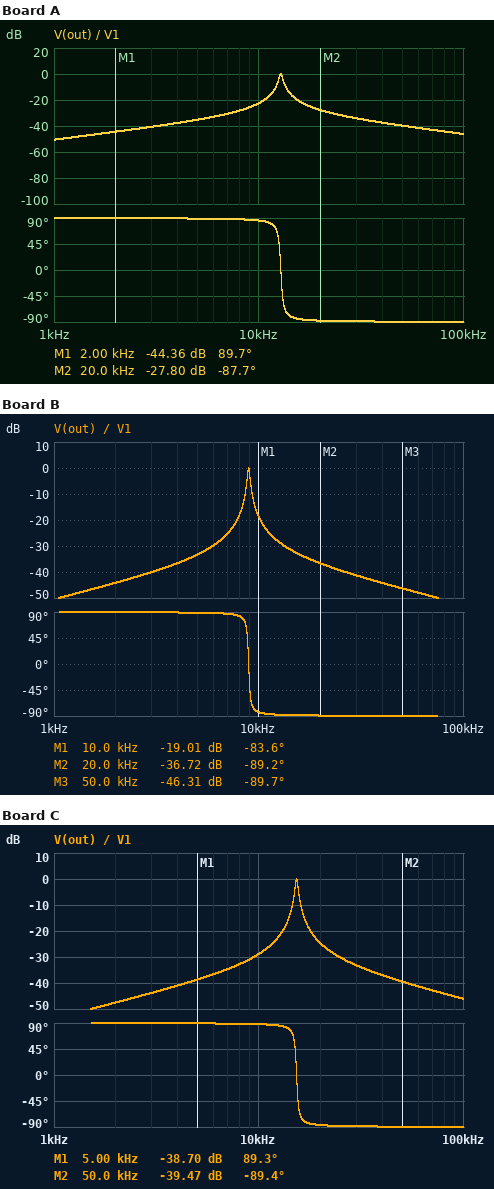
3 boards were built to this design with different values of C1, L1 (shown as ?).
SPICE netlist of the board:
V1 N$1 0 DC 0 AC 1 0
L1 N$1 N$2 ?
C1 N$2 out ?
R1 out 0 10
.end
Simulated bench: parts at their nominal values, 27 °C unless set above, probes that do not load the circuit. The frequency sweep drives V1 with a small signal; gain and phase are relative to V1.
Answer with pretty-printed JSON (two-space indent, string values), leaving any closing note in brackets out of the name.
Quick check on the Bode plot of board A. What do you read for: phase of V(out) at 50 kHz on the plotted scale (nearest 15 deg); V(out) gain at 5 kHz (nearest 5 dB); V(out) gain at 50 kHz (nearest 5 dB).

{
  "phase of V(out) at 50 kHz on the plotted scale": "-90 deg",
  "V(out) gain at 5 kHz": "-35 dB",
  "V(out) gain at 50 kHz": "-40 dB"
}
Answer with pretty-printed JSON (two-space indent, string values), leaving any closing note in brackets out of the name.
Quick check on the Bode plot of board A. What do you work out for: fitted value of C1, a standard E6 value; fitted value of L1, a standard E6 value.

{
  "fitted value of C1, a standard E6 value": "47 nF",
  "fitted value of L1, a standard E6 value": "3.3 mH"
}
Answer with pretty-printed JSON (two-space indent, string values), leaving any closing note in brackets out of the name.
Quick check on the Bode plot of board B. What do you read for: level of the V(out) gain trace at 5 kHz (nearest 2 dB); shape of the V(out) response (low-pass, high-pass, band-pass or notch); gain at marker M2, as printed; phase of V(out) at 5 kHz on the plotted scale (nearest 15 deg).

{
  "level of the V(out) gain trace at 5 kHz": "-34 dB",
  "shape of the V(out) response": "band-pass",
  "gain at marker M2, as printed": "-36.72 dB",
  "phase of V(out) at 5 kHz on the plotted scale": "90 deg"
}
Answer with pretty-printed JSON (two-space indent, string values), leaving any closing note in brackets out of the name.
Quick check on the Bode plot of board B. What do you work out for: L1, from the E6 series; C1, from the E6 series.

{
  "L1, from the E6 series": "6.8 mH",
  "C1, from the E6 series": "47 nF"
}
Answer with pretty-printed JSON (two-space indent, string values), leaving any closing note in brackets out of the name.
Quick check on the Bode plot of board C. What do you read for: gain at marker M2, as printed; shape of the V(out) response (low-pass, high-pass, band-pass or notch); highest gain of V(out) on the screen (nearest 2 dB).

{
  "gain at marker M2, as printed": "-39.47 dB",
  "shape of the V(out) response": "band-pass",
  "highest gain of V(out) on the screen": "0 dB"
}
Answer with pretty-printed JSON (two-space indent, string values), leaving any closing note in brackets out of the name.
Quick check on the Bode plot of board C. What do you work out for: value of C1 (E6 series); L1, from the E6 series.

{
  "value of C1": "33 nF",
  "L1, from the E6 series": "3.3 mH"
}
